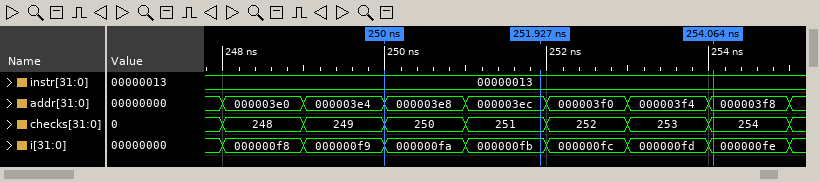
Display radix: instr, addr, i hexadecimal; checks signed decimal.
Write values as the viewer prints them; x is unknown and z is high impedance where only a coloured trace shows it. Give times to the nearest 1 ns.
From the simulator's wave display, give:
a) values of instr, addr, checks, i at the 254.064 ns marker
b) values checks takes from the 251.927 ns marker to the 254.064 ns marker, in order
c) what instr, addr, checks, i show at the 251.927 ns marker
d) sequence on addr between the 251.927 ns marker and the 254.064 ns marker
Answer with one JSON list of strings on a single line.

["instr=00000013, addr=000003f8, checks=254, i=000000fe", "251, 252, 253, 254", "instr=00000013, addr=000003ec, checks=251, i=000000fb", "000003ec, 000003f0, 000003f4, 000003f8"]
